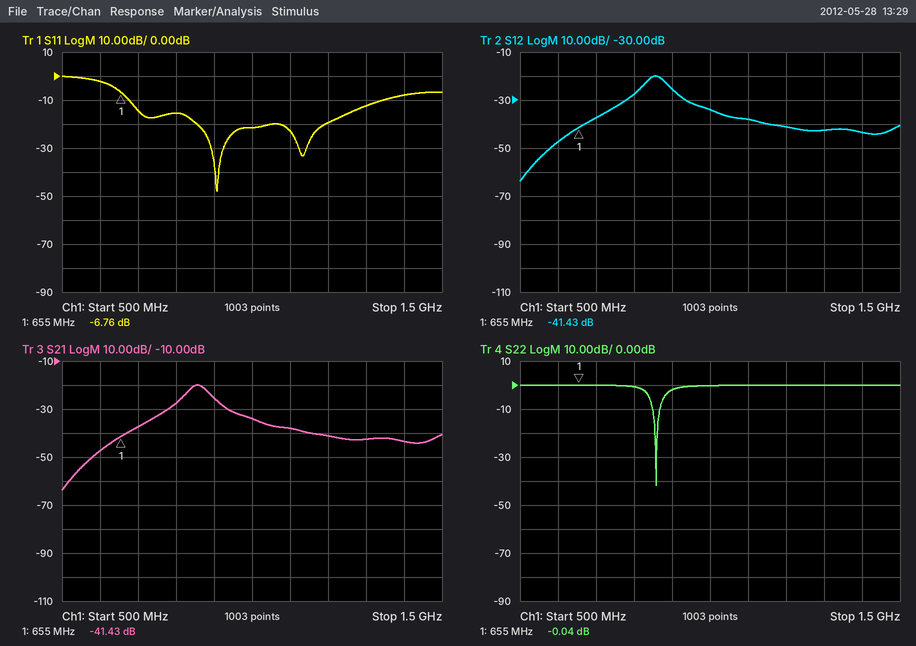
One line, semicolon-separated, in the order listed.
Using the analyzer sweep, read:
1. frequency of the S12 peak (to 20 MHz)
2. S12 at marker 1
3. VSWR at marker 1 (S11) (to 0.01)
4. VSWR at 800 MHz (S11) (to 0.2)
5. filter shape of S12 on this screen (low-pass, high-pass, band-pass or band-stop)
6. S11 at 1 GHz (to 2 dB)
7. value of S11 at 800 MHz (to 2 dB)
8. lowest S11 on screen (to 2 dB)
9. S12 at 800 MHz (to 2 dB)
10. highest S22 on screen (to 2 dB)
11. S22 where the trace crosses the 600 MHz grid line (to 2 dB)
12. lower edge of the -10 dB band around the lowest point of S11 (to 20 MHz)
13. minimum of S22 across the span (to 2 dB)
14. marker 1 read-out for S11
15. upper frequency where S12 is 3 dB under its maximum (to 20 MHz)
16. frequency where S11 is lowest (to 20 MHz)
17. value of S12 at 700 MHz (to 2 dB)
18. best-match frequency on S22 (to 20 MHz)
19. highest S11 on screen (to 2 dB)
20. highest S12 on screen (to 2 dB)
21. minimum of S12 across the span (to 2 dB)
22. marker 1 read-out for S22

860 MHz; -41.43 dB; 2.70; 1.4; band-pass; -22 dB; -16 dB; -48 dB; -28 dB; 0 dB; 0 dB; 680 MHz; -42 dB; -6.76 dB; 880 MHz; 900 MHz; -38 dB; 860 MHz; 0 dB; -20 dB; -64 dB; -0.04 dB
